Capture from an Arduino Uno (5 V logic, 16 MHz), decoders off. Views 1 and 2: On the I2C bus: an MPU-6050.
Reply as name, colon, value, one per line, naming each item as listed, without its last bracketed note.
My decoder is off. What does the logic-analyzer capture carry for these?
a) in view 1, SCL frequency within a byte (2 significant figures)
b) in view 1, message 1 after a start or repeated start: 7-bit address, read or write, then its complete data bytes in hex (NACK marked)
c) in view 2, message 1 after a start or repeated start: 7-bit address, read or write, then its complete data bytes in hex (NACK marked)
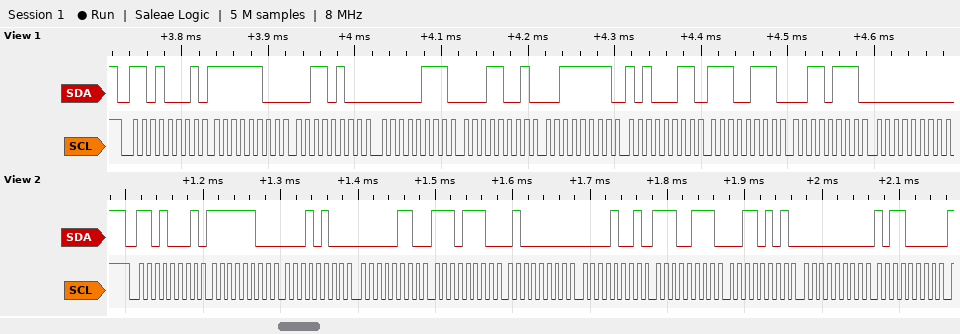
in view 1, SCL frequency within a byte: 100 kHz
in view 1, message 1 after a start or repeated start: 7-bit address, read or write, then its complete data bytes in hex: 0x68 read: FC 34 07 19 3F A3 E7 37 00
in view 2, message 1 after a start or repeated start: 7-bit address, read or write, then its complete data bytes in hex: 0x68 read: FC 14 06 EE 40 09 E7 35 00 B0
